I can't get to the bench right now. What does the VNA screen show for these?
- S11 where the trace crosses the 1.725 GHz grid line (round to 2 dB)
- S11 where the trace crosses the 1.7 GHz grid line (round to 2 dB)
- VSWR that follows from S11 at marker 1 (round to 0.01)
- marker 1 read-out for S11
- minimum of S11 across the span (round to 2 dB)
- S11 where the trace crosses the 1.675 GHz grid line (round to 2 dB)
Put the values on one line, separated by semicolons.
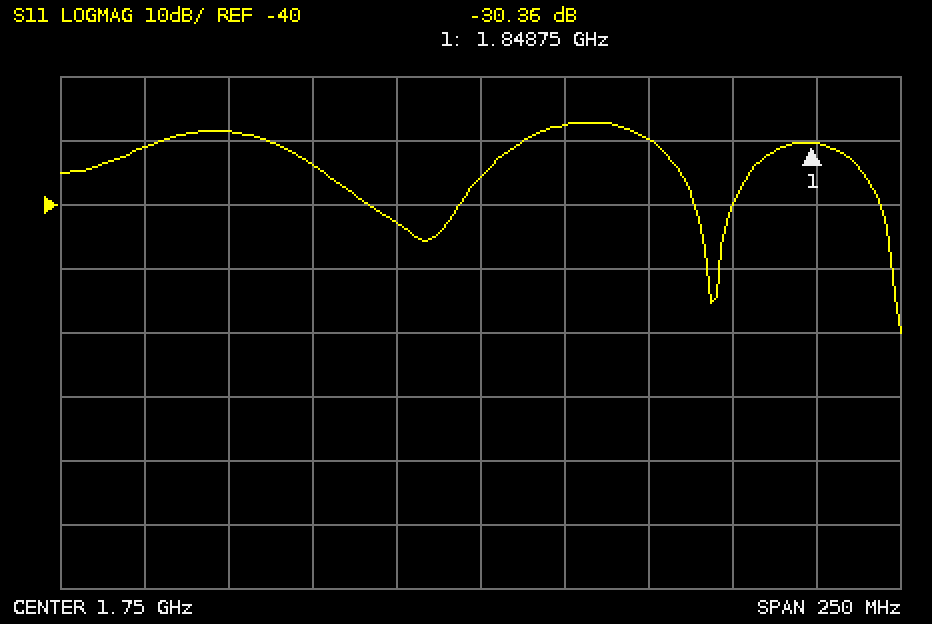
-42 dB; -34 dB; 1.06; -30.36 dB; -60 dB; -28 dB
